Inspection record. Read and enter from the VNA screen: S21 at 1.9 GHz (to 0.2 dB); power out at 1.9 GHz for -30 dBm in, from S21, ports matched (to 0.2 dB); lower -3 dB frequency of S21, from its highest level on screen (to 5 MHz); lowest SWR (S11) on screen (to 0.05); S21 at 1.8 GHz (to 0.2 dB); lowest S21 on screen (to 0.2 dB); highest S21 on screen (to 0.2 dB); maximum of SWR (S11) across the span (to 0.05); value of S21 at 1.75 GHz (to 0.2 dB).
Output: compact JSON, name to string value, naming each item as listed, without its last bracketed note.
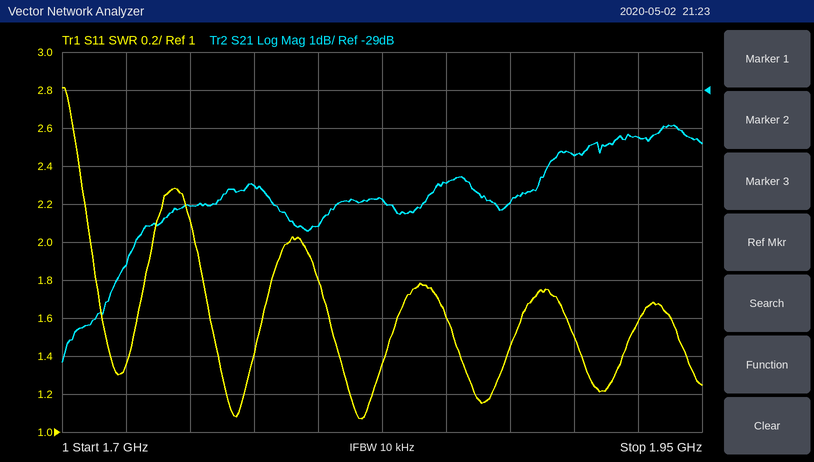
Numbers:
{"S21 at 1.9 GHz": "-30.8 dB", "power out at 1.9 GHz for -30 dBm in, from S21, ports matched": "-60.8 dBm", "lower -3 dB frequency of S21, from its highest level on screen": "1.730 GHz", "lowest SWR (S11) on screen": "1.05", "S21 at 1.8 GHz": "-32.6 dB", "lowest S21 on screen": "-36.2 dB", "highest S21 on screen": "-30.0 dB", "maximum of SWR (S11) across the span": "2.80", "value of S21 at 1.75 GHz": "-32.0 dB"}
